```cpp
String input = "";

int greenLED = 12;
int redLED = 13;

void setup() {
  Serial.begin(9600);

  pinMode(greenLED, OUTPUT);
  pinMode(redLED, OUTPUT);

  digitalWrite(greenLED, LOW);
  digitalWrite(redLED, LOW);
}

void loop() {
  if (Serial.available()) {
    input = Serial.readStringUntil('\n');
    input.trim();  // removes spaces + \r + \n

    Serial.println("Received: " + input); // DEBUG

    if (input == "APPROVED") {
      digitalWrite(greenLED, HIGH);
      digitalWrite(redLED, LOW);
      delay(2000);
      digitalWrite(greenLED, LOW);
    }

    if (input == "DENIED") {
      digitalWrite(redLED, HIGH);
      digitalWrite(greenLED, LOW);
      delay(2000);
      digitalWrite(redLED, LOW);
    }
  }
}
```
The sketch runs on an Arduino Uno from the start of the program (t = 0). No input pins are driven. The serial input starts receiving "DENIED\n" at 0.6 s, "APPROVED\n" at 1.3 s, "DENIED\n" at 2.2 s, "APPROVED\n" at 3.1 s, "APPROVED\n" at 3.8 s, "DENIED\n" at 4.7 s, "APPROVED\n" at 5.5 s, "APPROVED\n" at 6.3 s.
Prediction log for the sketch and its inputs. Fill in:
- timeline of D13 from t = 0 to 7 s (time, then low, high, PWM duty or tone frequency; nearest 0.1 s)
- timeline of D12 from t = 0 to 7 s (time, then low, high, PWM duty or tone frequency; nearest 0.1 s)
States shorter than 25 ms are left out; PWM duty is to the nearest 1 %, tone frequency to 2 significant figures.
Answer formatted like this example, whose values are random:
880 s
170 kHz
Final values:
0 s low; 0.6 s high; 2.6 s low; 4.6 s high; 6.6 s low
0 s low; 2.6 s high; 4.6 s low; 6.6 s high
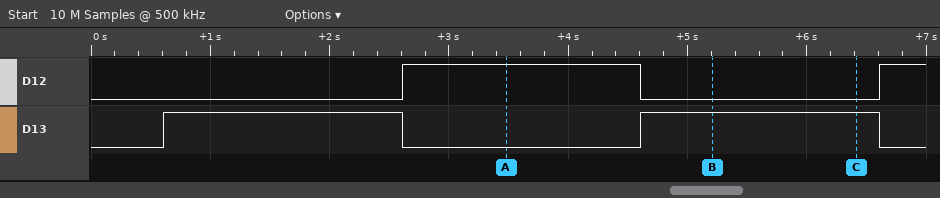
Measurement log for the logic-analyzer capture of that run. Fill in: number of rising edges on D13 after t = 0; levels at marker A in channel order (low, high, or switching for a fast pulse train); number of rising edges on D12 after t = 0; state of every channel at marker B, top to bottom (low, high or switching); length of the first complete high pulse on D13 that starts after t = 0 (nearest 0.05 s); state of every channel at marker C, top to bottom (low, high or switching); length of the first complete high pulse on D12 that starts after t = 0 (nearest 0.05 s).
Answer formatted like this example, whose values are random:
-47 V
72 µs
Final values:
2
D12 high, D13 low
2
D12 low, D13 high
2.00 s
D12 low, D13 high
2.00 s
